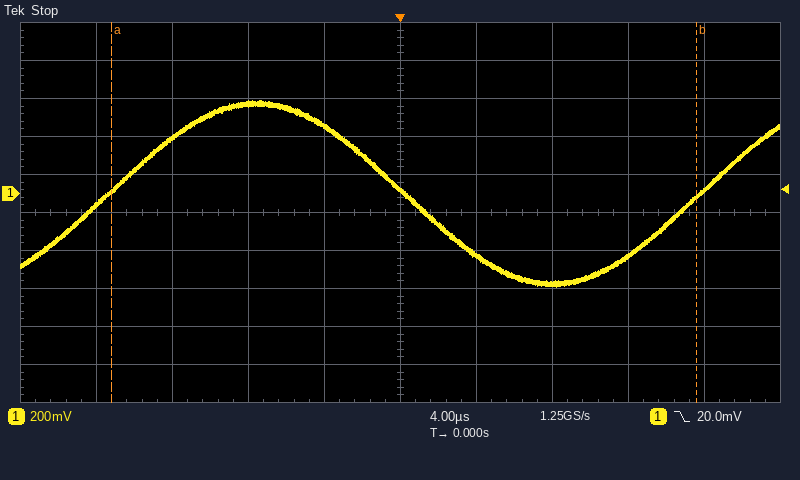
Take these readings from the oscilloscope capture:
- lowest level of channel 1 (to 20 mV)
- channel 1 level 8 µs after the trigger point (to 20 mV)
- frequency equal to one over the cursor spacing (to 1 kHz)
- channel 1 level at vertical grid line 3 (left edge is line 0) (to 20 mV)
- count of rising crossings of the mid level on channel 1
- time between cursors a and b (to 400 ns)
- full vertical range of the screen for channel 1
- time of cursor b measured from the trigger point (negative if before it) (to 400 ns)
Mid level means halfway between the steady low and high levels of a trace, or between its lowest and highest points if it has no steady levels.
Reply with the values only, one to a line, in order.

-480 mV
-480 mV
32 kHz
480 mV
2
30.8 µs
2 V
+15.6 µs
